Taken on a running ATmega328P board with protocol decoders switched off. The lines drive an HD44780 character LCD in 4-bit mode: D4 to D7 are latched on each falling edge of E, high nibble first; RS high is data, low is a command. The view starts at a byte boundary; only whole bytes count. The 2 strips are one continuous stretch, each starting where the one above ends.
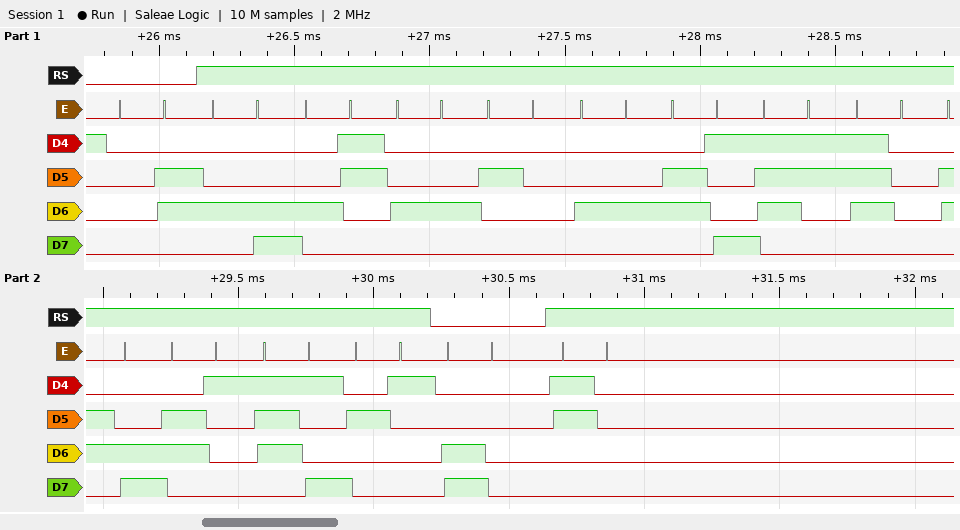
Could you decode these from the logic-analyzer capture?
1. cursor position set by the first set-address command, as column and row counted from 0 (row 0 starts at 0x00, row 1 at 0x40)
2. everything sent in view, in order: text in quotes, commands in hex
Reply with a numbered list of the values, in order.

1. column 0, row 1
2. 0x06 "LCD Display!" 0xC0 "0"
